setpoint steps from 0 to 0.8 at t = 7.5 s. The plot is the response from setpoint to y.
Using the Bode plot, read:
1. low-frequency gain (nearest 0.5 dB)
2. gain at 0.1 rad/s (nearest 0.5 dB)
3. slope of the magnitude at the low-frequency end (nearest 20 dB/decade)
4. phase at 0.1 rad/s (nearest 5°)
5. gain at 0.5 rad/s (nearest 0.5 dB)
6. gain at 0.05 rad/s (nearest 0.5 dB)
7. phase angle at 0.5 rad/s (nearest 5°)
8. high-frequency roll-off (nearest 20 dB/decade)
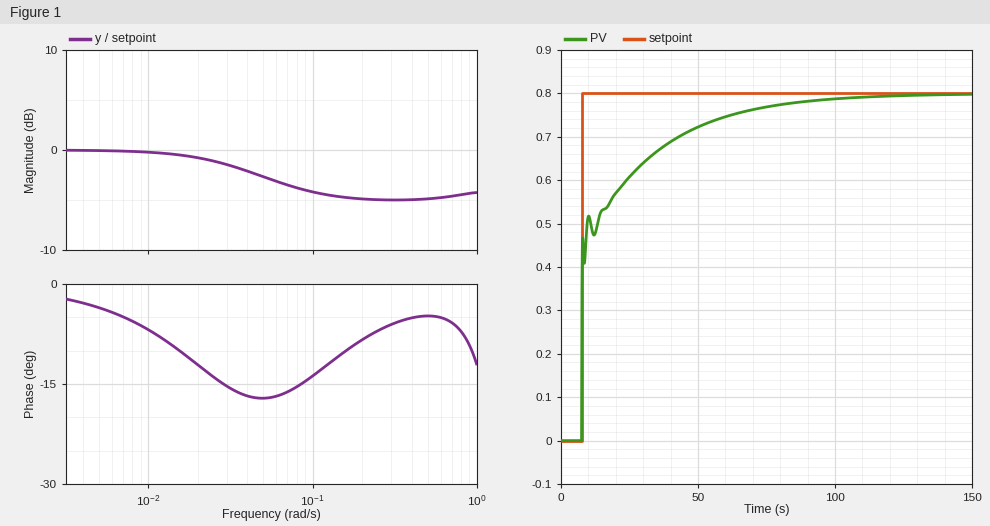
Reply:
0.0 dB
-4.0 dB
0 dB/decade
-15°
-5.0 dB
-2.5 dB
-5°
0 dB/decade
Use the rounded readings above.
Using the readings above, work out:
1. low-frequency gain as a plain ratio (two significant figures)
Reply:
1.0
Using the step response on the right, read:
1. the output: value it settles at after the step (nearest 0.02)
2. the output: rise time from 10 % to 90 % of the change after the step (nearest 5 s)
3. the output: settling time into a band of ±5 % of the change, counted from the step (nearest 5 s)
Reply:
0.80
40 s
60 s
